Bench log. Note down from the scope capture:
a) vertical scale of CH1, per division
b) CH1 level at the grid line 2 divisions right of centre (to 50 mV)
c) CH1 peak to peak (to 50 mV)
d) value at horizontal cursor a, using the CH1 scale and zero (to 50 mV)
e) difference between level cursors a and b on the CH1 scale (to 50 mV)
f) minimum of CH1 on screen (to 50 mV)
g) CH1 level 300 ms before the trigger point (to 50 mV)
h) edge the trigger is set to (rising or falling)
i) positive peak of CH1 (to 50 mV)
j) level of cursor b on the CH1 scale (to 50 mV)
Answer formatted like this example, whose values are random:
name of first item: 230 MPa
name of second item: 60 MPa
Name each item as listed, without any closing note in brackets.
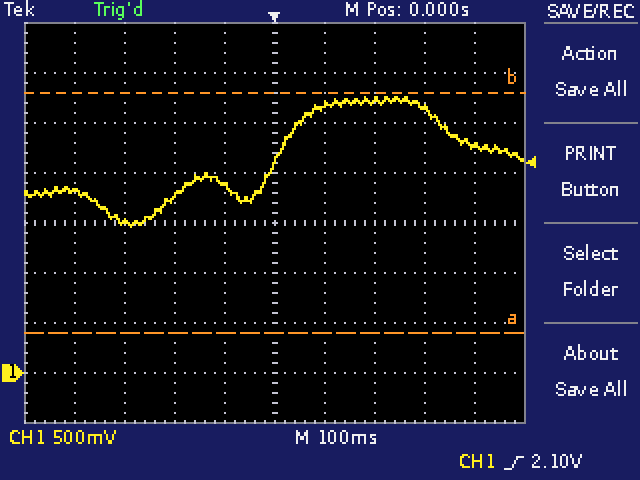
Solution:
vertical scale of CH1, per division: 500 mV
CH1 level at the grid line 2 divisions right of centre: 2.70 V
CH1 peak to peak: 1.30 V
value at horizontal cursor a, using the CH1 scale and zero: 400 mV
difference between level cursors a and b on the CH1 scale: 2.40 V
minimum of CH1 on screen: 1.45 V
CH1 level 300 ms before the trigger point: 1.50 V
edge the trigger is set to: rising
positive peak of CH1: 2.75 V
level of cursor b on the CH1 scale: 2.80 V
